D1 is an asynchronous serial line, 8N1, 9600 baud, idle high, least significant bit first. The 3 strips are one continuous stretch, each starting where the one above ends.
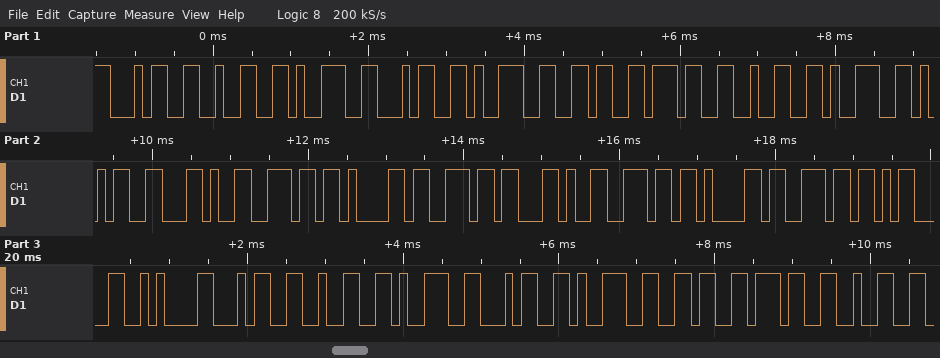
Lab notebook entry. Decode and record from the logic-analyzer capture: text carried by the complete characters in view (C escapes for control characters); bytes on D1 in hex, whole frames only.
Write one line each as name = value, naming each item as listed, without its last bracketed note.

text carried by the complete characters in view = "4294967295,nan,nan\r\n42949672"
bytes on D1 in hex, whole frames only = 34 32 39 34 39 36 37 32 39 35 2C 6E 61 6E 2C 6E 61 6E 0D 0A 34 32 39 34 39 36 37 32
